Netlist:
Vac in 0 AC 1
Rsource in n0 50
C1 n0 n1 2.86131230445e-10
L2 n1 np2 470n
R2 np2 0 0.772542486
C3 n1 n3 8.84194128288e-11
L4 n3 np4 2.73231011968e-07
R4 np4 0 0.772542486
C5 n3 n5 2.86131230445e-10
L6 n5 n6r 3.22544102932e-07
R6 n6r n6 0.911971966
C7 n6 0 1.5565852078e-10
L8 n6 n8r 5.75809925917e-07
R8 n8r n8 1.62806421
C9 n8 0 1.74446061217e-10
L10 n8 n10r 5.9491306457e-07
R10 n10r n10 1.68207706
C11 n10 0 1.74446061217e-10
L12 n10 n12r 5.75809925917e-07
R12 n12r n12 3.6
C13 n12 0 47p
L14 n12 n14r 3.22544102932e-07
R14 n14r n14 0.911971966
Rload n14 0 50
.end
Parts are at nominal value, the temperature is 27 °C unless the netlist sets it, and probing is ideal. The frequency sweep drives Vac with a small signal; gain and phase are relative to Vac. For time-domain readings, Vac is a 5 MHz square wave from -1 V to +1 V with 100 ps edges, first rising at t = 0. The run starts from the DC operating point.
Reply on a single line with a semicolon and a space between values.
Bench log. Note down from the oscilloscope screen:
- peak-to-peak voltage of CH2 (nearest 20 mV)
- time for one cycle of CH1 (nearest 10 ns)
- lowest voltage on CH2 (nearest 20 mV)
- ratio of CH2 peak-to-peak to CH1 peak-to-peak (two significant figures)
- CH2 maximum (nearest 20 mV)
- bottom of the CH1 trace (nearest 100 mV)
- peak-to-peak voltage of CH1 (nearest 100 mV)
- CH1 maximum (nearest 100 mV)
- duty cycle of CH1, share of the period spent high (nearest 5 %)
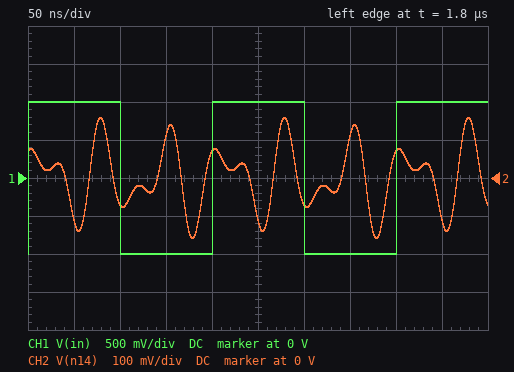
320 mV; 200 ns; -160 mV; 0.16; 160 mV; -1.0 V; 2.0 V; 1.0 V; 50 %
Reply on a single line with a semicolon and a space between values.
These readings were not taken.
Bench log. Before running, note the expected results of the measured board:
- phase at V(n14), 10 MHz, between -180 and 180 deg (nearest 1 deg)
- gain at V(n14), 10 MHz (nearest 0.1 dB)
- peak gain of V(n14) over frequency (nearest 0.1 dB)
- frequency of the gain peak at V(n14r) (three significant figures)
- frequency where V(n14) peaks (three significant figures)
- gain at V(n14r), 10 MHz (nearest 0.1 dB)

-164 deg; -26.4 dB; -7.4 dB; 21.6 MHz; 21.6 MHz; -26.2 dB
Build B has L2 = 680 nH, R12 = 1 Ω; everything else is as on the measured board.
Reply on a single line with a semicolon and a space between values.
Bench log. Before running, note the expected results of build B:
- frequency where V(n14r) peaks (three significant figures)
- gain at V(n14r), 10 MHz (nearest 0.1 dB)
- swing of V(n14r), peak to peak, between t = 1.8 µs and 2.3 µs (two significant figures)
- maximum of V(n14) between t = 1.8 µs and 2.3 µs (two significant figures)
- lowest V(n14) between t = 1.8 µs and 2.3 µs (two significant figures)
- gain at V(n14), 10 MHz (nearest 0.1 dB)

21.7 MHz; -21.6 dB; 310 mV; 150 mV; -150 mV; -21.7 dB
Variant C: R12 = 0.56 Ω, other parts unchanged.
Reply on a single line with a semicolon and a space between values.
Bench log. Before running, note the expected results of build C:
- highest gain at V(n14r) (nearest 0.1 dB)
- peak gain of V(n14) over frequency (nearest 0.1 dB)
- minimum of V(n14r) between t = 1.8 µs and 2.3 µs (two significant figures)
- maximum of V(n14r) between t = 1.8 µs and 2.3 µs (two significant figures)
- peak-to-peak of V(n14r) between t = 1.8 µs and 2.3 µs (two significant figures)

-7.1 dB; -7.2 dB; -170 mV; 170 mV; 330 mV
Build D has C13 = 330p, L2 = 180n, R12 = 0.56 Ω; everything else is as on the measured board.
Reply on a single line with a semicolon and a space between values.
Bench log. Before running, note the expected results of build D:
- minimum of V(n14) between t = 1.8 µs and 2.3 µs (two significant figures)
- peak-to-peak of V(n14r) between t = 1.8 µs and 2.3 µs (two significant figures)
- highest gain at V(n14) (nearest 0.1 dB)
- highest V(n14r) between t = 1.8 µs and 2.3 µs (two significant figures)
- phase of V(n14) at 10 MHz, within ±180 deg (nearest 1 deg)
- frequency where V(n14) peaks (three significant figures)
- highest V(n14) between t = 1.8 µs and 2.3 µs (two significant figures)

-95 mV; 190 mV; -8.3 dB; 97 mV; 162 deg; 22.9 MHz; 95 mV
